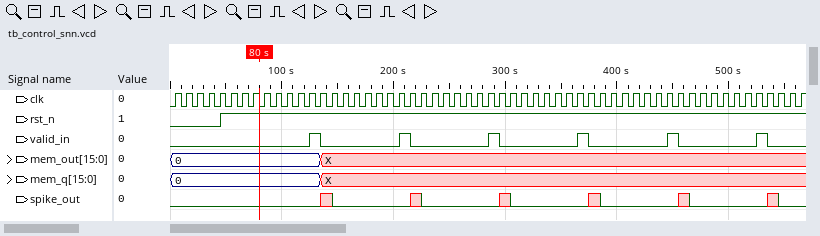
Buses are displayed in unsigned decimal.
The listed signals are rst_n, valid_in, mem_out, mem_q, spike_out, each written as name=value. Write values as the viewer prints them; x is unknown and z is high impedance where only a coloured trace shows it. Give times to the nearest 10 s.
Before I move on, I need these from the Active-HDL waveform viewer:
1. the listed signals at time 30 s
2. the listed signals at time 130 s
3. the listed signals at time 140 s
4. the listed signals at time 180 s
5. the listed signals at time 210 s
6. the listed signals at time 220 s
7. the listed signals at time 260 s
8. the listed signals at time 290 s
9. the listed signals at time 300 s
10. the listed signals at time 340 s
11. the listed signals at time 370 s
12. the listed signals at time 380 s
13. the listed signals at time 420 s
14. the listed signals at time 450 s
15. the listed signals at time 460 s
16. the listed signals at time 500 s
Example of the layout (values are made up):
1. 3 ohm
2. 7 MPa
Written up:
1. rst_n=0, valid_in=0, mem_out=0, mem_q=0, spike_out=0
2. rst_n=1, valid_in=1, mem_out=0, mem_q=0, spike_out=0
3. rst_n=1, valid_in=0, mem_out=X, mem_q=X, spike_out=x
4. rst_n=1, valid_in=0, mem_out=X, mem_q=X, spike_out=0
5. rst_n=1, valid_in=1, mem_out=X, mem_q=X, spike_out=0
6. rst_n=1, valid_in=0, mem_out=X, mem_q=X, spike_out=x
7. rst_n=1, valid_in=0, mem_out=X, mem_q=X, spike_out=0
8. rst_n=1, valid_in=1, mem_out=X, mem_q=X, spike_out=0
9. rst_n=1, valid_in=0, mem_out=X, mem_q=X, spike_out=x
10. rst_n=1, valid_in=0, mem_out=X, mem_q=X, spike_out=0
11. rst_n=1, valid_in=1, mem_out=X, mem_q=X, spike_out=0
12. rst_n=1, valid_in=0, mem_out=X, mem_q=X, spike_out=x
13. rst_n=1, valid_in=0, mem_out=X, mem_q=X, spike_out=0
14. rst_n=1, valid_in=1, mem_out=X, mem_q=X, spike_out=0
15. rst_n=1, valid_in=0, mem_out=X, mem_q=X, spike_out=x
16. rst_n=1, valid_in=0, mem_out=X, mem_q=X, spike_out=0
